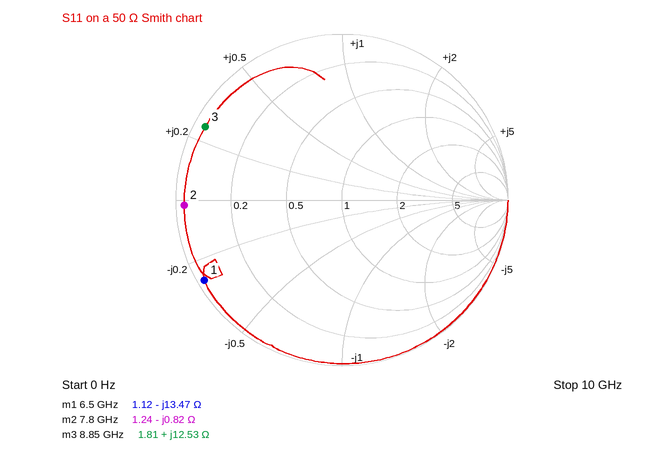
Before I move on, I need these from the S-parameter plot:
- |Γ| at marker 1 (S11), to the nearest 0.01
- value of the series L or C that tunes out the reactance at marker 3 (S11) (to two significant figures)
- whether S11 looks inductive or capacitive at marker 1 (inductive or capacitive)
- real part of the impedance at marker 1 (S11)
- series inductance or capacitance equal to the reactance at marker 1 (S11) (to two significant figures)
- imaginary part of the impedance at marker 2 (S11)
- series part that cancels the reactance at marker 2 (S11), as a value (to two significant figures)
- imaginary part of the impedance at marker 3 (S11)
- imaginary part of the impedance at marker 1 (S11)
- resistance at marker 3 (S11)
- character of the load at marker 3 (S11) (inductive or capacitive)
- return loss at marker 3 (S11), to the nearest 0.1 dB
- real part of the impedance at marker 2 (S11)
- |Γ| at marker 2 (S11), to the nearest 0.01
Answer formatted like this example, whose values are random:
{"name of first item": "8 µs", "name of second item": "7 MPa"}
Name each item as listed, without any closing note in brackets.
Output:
{"|Γ| at marker 1 (S11), to the nearest 0.01": "0.96", "value of the series L or C that tunes out the reactance at marker 3 (S11)": "1.4 pF", "whether S11 looks inductive or capacitive at marker 1": "capacitive", "real part of the impedance at marker 1": "1.12 Ω", "series inductance or capacitance equal to the reactance at marker 1 (S11)": "1.8 pF", "imaginary part of the impedance at marker 2": "-0.82 Ω", "series part that cancels the reactance at marker 2 (S11), as a value": "17 pH", "imaginary part of the impedance at marker 3": "+12.53 Ω", "imaginary part of the impedance at marker 1": "-13.47 Ω", "resistance at marker 3": "1.81 Ω", "character of the load at marker 3 (S11)": "inductive", "return loss at marker 3 (S11), to the nearest 0.1 dB": "0.6 dB", "real part of the impedance at marker 2": "1.24 Ω", "|Γ| at marker 2 (S11), to the nearest 0.01": "0.95"}
